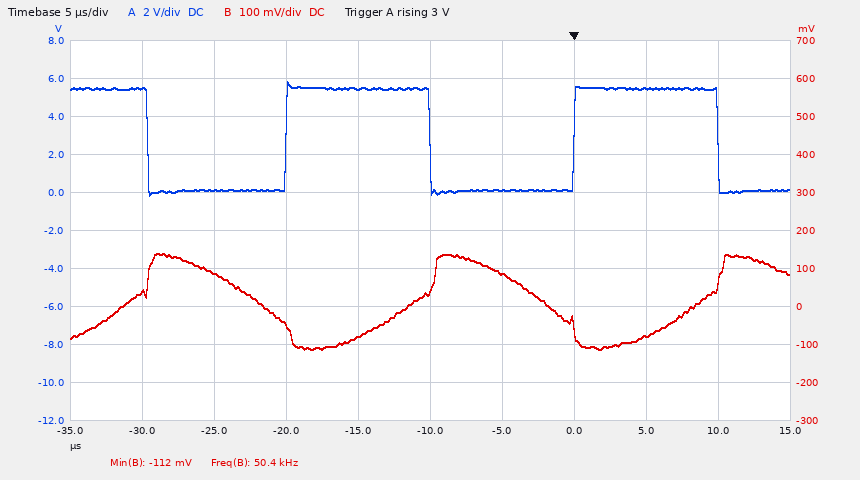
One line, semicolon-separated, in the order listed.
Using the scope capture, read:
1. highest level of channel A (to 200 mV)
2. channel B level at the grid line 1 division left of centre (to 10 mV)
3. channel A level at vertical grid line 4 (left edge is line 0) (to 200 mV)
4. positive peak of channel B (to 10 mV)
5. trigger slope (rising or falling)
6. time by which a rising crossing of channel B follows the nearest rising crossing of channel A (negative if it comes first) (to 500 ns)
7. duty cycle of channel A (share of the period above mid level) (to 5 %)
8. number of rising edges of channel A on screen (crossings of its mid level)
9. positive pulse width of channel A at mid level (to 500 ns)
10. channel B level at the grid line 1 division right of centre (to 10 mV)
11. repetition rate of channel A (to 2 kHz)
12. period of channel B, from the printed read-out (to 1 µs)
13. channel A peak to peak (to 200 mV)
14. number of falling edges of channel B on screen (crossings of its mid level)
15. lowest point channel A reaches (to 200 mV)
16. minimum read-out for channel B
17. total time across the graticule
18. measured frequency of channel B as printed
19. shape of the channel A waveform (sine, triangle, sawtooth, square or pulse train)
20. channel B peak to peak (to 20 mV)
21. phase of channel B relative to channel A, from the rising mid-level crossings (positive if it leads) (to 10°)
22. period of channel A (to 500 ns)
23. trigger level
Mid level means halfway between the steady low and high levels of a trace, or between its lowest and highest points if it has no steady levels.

5.8 V; -80 mV; 5.4 V; 140 mV; rising; +9.0 µs; 50 %; 2; 10.0 µs; 90 mV; 50 kHz; 20 µs; 6.0 V; 2; -200 mV; -112 mV; 50 µs; 50.4 kHz; square; 260 mV; -160°; 20.0 µs; 3 V
